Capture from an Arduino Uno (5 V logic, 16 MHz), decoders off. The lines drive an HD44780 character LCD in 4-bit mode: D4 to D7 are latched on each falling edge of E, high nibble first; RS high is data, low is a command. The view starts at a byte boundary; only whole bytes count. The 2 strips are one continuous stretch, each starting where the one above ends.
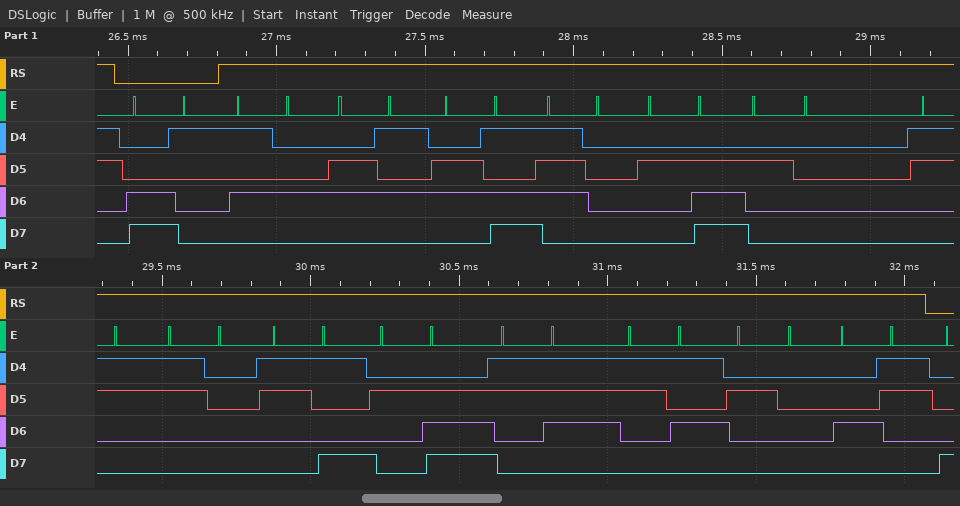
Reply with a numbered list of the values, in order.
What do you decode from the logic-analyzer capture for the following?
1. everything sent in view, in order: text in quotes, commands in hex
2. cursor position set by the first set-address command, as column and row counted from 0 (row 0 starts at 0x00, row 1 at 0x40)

1. 0xC1 "Temp. 309.75 C"
2. column 1, row 1
